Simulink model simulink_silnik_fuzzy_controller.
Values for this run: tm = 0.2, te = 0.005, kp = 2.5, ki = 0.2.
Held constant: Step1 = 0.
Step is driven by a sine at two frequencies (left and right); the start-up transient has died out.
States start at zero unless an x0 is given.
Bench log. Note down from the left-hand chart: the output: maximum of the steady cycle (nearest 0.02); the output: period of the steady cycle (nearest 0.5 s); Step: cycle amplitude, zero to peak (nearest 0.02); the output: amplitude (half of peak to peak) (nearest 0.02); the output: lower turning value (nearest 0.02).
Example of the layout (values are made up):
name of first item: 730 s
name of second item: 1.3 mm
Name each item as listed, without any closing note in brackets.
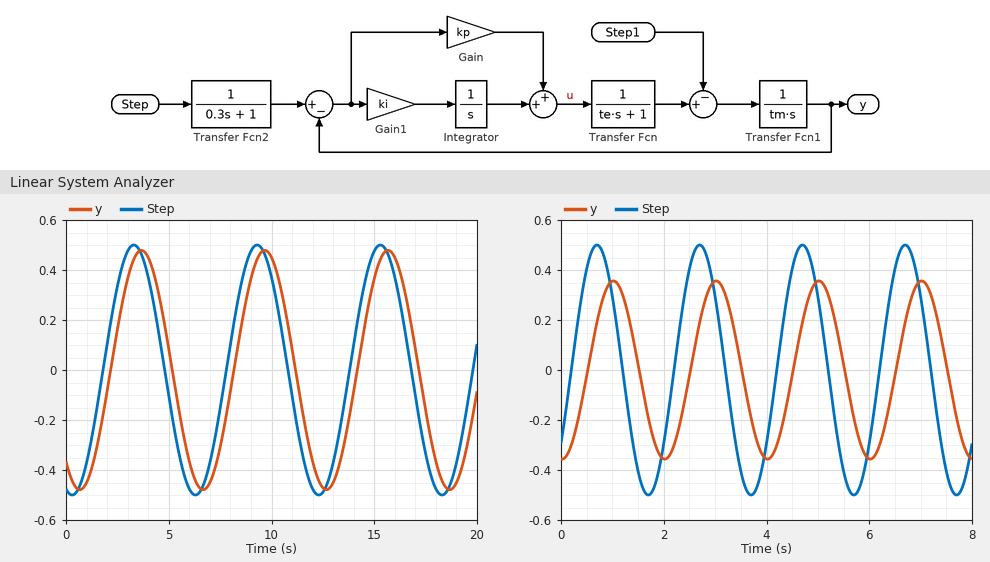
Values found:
the output: maximum of the steady cycle: 0.48
the output: period of the steady cycle: 6.0 s
Step: cycle amplitude, zero to peak: 0.50
the output: amplitude (half of peak to peak): 0.48
the output: lower turning value: -0.48
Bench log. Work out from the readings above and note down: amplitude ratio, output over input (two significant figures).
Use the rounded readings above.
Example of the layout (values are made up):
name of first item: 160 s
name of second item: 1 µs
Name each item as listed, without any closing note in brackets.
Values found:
amplitude ratio, output over input: 0.96
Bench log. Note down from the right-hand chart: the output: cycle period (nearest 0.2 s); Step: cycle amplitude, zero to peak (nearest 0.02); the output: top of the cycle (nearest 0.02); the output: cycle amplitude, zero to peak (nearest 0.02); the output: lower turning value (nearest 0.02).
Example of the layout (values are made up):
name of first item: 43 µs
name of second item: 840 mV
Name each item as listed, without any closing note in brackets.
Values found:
the output: cycle period: 2.0 s
Step: cycle amplitude, zero to peak: 0.50
the output: top of the cycle: 0.36
the output: cycle amplitude, zero to peak: 0.36
the output: lower turning value: -0.36
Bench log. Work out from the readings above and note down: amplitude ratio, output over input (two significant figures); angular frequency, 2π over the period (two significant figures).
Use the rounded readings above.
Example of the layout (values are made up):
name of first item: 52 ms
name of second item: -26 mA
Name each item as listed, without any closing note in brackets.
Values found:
amplitude ratio, output over input: 0.72
angular frequency, 2π over the period: 3.1 rad/s
